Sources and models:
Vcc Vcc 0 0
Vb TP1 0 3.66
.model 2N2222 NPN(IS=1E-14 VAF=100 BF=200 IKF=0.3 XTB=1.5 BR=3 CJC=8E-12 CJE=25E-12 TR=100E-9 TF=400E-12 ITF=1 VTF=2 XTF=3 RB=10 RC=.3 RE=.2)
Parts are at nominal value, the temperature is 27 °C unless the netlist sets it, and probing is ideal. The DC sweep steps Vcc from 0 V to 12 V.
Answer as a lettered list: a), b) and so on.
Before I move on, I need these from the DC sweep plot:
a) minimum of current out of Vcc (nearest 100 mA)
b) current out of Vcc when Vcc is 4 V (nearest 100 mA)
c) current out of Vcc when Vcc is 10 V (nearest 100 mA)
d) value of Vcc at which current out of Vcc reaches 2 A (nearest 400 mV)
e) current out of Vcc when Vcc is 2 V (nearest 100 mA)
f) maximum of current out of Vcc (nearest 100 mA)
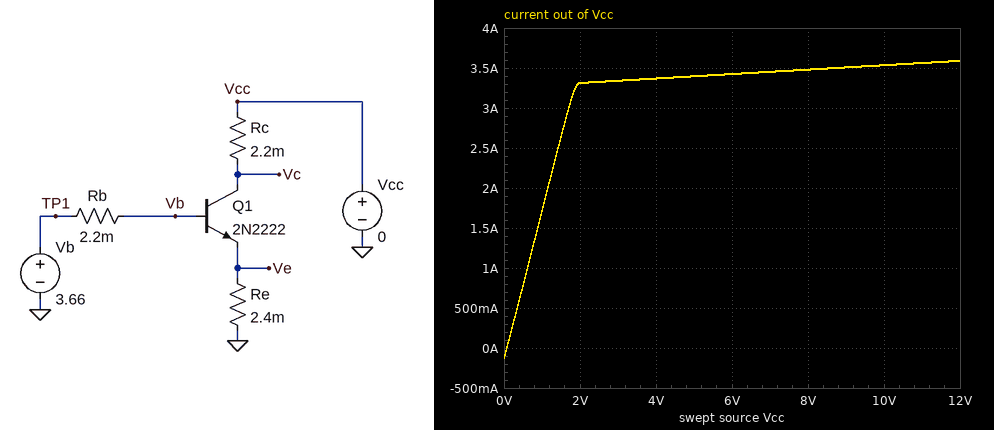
a) -100 mA
b) 3.4 A
c) 3.5 A
d) 1.2 V
e) 3.3 A
f) 3.6 A
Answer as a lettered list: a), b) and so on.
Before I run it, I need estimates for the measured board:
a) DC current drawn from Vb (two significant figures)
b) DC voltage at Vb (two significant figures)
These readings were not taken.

a) 280 mA
b) 3.7 V
